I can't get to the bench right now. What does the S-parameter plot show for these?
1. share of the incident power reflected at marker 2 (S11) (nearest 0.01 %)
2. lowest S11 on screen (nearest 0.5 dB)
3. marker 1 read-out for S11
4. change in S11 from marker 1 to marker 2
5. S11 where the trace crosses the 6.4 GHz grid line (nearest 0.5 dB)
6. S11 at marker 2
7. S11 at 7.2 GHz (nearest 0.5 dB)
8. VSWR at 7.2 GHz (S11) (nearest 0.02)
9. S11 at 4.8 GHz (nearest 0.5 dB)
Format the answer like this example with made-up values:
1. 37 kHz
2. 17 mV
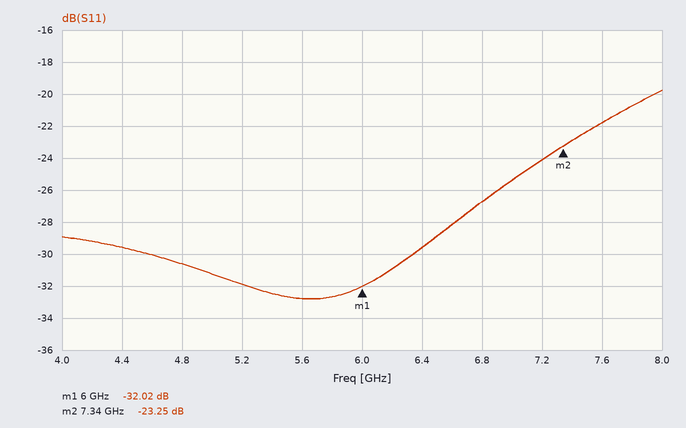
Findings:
1. 0.47 %
2. -33.0 dB
3. -32.02 dB
4. 8.77 dB
5. -29.5 dB
6. -23.25 dB
7. -24.0 dB
8. 1.14
9. -30.5 dB
